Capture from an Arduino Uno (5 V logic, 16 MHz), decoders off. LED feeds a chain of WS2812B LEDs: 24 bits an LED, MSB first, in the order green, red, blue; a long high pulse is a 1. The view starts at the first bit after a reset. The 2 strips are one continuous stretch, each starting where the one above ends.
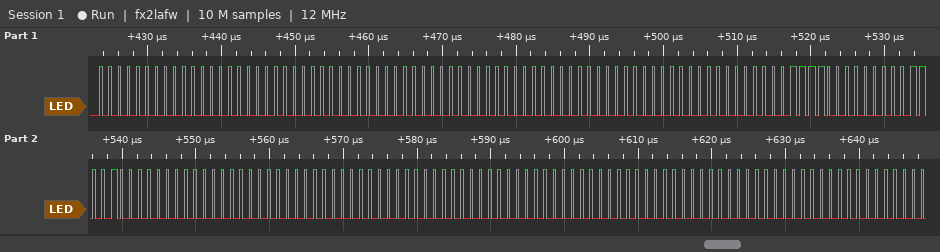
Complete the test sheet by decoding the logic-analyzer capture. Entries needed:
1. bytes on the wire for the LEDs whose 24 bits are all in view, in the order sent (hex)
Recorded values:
00 00 00 00 00 00 00 00 00 1E 00 C8 00 00 00 00 00 00 00 00 00
